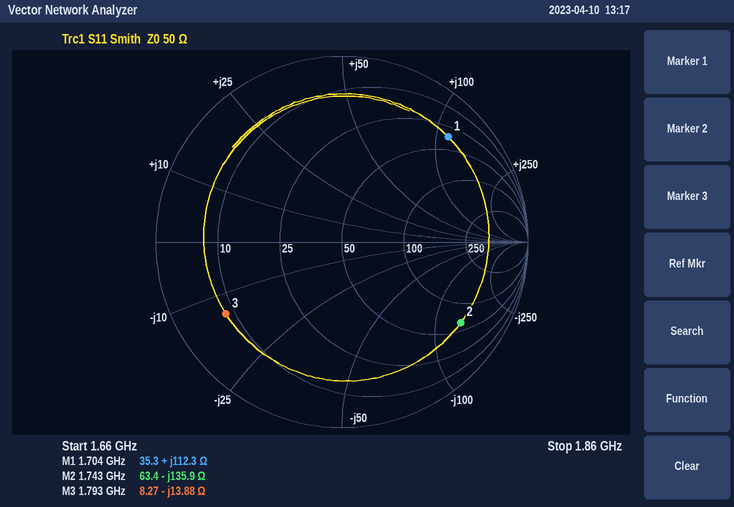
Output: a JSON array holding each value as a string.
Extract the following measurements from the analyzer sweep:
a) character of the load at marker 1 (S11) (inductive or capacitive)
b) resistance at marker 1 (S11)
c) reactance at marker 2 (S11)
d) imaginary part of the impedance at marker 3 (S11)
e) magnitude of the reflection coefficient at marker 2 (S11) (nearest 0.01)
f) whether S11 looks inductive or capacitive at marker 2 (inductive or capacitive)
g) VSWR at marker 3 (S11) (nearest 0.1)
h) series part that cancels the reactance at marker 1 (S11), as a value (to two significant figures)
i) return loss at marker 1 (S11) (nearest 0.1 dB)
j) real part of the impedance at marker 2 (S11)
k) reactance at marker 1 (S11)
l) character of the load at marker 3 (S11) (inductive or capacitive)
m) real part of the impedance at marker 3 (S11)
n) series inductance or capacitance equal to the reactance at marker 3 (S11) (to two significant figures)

["inductive", "35.3 Ω", "-135.9 Ω", "-13.88 Ω", "0.77", "capacitive", "6.5", "830 fF", "1.9 dB", "63.4 Ω", "+112.3 Ω", "capacitive", "8.27 Ω", "6.4 pF"]
